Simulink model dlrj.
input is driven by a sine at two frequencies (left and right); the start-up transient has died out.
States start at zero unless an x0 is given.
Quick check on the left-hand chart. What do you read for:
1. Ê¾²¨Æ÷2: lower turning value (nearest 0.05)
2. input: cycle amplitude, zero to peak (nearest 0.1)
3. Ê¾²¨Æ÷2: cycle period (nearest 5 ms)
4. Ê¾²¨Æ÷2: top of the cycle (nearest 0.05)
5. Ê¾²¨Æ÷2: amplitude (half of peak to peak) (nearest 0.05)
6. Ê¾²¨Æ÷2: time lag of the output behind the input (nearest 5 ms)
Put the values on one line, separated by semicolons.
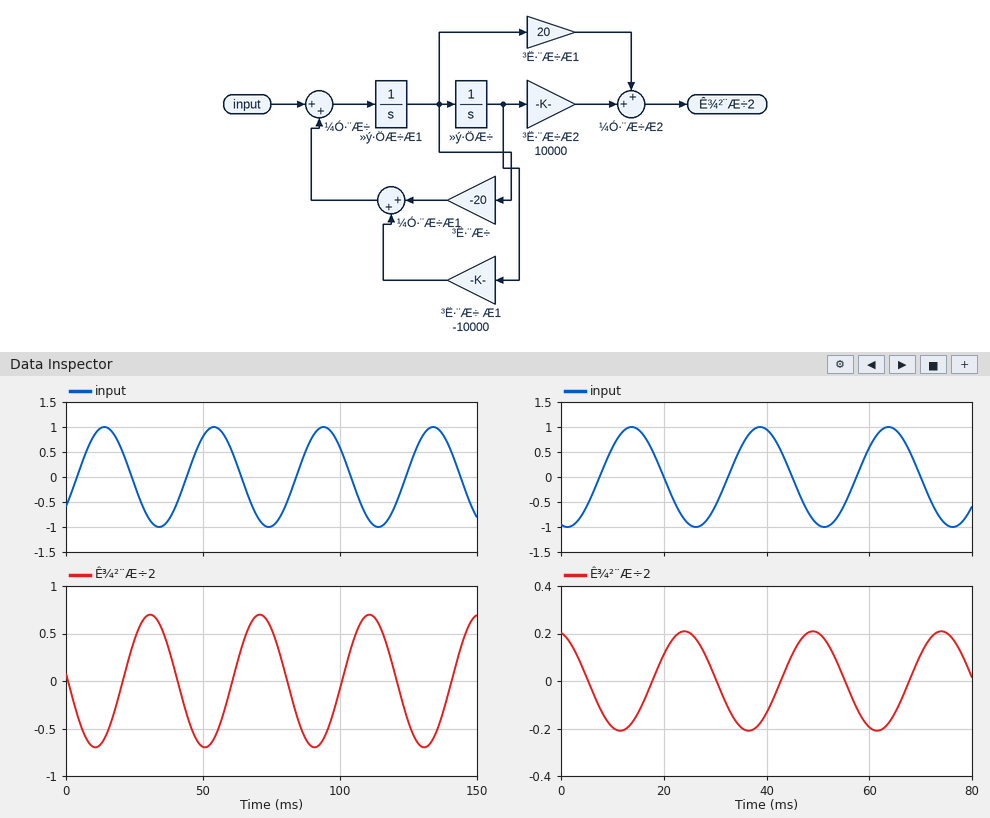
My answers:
-0.70; 1.0; 40 ms; 0.70; 0.70; 15 ms
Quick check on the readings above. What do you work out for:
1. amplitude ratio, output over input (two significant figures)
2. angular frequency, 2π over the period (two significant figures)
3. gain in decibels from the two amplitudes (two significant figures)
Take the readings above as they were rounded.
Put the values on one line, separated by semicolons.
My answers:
0.70; 0.16 rad/ms; -3.1 dB
